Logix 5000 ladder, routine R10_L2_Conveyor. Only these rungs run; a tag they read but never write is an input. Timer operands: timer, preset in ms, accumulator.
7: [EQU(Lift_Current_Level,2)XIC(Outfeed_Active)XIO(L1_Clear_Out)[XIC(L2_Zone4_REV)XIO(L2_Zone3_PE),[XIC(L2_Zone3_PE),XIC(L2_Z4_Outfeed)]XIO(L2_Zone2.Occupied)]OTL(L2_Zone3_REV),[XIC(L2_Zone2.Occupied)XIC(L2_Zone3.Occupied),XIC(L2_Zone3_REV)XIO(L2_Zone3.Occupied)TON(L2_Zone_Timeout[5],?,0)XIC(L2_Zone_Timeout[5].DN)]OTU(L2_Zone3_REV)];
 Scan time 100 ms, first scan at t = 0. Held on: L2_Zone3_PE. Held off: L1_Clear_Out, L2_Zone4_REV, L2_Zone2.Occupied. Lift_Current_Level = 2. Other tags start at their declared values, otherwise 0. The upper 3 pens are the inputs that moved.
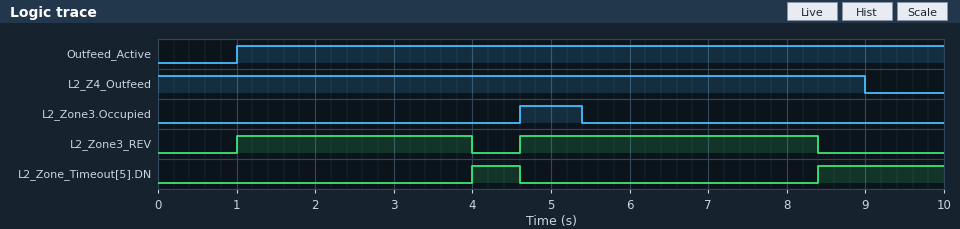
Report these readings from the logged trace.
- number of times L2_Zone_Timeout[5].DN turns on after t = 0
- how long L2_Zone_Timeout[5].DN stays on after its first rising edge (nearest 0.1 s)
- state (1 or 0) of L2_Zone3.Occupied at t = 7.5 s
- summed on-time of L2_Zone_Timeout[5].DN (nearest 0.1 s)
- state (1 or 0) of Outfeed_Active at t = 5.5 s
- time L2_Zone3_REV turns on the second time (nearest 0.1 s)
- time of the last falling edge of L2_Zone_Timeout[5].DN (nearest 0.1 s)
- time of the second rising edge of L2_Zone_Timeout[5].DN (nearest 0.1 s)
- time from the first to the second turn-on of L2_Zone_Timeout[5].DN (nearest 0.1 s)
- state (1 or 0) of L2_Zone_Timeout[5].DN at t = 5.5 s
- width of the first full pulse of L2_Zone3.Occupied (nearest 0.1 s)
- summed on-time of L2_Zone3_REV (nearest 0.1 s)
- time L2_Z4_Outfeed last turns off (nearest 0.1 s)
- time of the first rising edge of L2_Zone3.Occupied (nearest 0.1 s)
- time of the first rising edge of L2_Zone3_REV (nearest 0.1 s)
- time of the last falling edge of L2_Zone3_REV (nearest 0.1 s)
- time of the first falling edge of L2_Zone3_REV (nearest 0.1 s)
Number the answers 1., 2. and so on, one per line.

1. 2
2. 0.6 s
3. 0
4. 2.2 s
5. 1
6. 4.6 s
7. 4.6 s
8. 8.4 s
9. 4.4 s
10. 0
11. 0.8 s
12. 6.8 s
13. 9.0 s
14. 4.6 s
15. 1.0 s
16. 8.4 s
17. 4.0 s
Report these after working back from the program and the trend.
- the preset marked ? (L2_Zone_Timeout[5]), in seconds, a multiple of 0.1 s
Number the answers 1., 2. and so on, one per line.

1. 3.0 s
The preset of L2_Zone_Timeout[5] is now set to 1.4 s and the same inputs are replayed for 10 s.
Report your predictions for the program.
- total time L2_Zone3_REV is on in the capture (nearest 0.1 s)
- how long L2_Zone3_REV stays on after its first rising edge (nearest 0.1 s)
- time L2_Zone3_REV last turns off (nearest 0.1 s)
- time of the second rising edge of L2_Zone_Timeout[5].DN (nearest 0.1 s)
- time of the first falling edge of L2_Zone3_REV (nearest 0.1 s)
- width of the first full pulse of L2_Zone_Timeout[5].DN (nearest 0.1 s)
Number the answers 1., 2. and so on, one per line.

1. 3.6 s
2. 1.4 s
3. 6.8 s
4. 6.8 s
5. 2.4 s
6. 2.2 s
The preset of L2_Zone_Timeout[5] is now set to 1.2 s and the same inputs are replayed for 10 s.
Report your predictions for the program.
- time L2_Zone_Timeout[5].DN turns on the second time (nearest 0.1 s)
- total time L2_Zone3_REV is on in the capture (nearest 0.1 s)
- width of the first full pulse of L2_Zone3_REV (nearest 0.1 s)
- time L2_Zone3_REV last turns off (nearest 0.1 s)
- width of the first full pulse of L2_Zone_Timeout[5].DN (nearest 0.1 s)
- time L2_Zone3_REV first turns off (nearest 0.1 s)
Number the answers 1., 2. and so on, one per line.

1. 6.6 s
2. 3.2 s
3. 1.2 s
4. 6.6 s
5. 2.4 s
6. 2.2 s
